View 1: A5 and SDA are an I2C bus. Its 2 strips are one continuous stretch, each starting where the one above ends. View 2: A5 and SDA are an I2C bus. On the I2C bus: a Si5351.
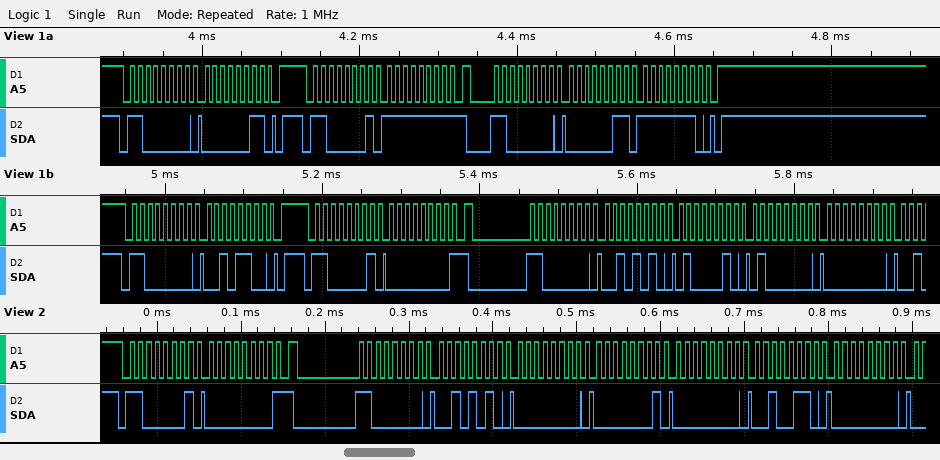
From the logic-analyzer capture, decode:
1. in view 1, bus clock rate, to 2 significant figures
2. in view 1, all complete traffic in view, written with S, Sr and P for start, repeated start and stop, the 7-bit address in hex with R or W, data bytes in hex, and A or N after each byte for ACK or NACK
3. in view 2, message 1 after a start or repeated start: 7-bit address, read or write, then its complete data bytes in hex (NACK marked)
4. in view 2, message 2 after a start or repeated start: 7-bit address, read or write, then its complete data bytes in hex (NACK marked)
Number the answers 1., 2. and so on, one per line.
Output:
1. 100 kHz
2. S 60W A 03 A P S 60R A FF N Sr 60W A 03 A FE A P S 60W A 2C A P S 60R A 00 N Sr 60W A 2A A 42 A 40 A 00 A
3. 0x60 read: 00 NACK
4. 0x60 write: 2A 00 01 00 26 00
